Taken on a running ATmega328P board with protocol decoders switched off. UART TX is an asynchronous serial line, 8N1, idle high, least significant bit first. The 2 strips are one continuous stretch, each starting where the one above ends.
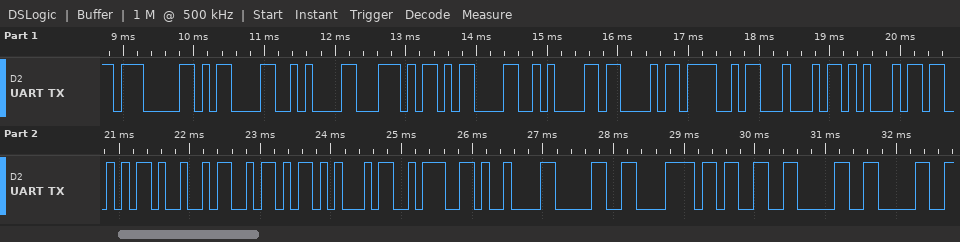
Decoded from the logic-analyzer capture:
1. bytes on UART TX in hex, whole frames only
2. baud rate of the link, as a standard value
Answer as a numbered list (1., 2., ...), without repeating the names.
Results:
1. 07 0D 0A 5C 0D 0A 43 4F 44 45 53 49 5A 45 3A 09 30 78 33 30 30
2. 9600 baud
